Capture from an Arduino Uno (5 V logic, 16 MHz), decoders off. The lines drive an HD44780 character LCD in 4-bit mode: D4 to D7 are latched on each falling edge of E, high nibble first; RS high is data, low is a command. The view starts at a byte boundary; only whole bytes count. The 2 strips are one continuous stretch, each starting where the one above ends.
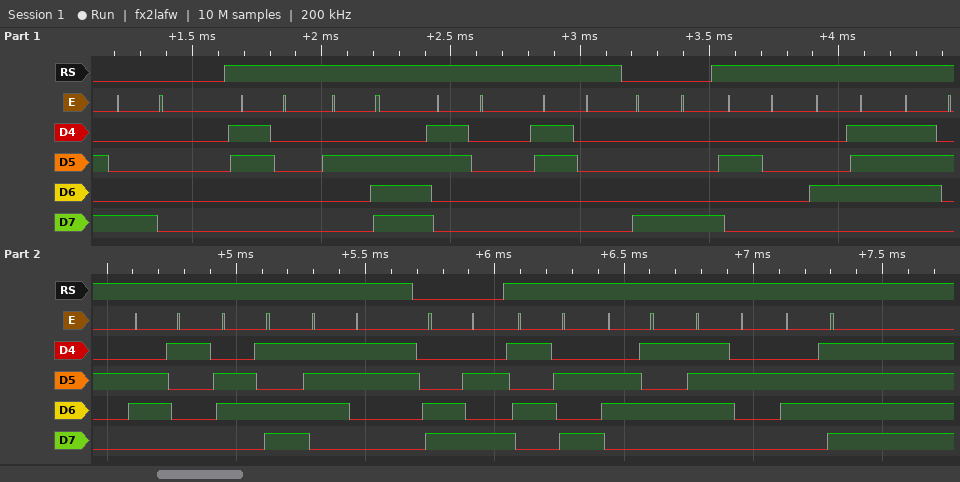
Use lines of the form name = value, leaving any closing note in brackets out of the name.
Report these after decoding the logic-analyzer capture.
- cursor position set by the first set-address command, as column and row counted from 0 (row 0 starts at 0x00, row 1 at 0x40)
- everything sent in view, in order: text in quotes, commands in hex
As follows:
cursor position set by the first set-address command, as column and row counted from 0 = column 0, row 0
everything sent in view, in order: text in quotes, commands in hex = 0x80 "0.00" 0x88 " Grams" 0xCA "Zero"
